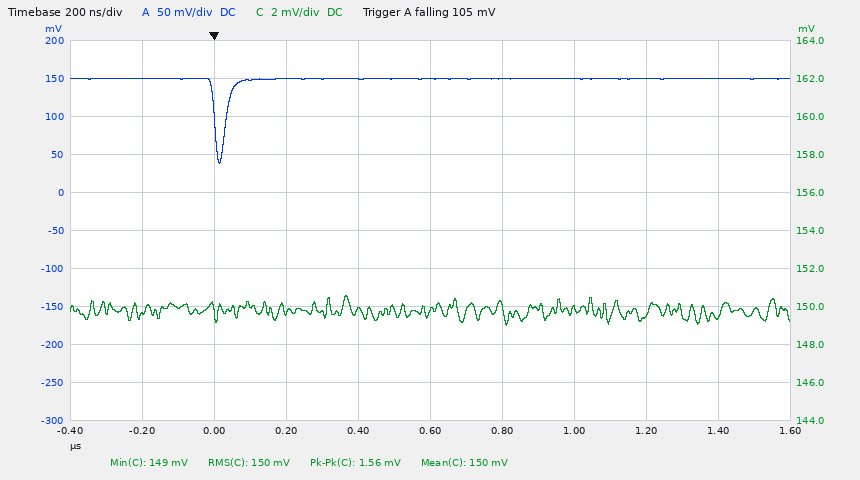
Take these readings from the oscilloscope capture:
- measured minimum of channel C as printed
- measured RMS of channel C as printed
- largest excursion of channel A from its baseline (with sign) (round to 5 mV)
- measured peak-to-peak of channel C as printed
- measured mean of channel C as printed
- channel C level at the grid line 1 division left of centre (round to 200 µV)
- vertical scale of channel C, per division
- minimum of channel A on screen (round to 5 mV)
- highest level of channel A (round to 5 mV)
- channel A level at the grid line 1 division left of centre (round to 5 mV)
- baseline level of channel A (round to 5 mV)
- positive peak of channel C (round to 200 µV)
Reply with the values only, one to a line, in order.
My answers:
149 mV
150 mV
-110 mV
1.56 mV
150 mV
149.8 mV
2 mV
40 mV
150 mV
150 mV
150 mV
150.6 mV
